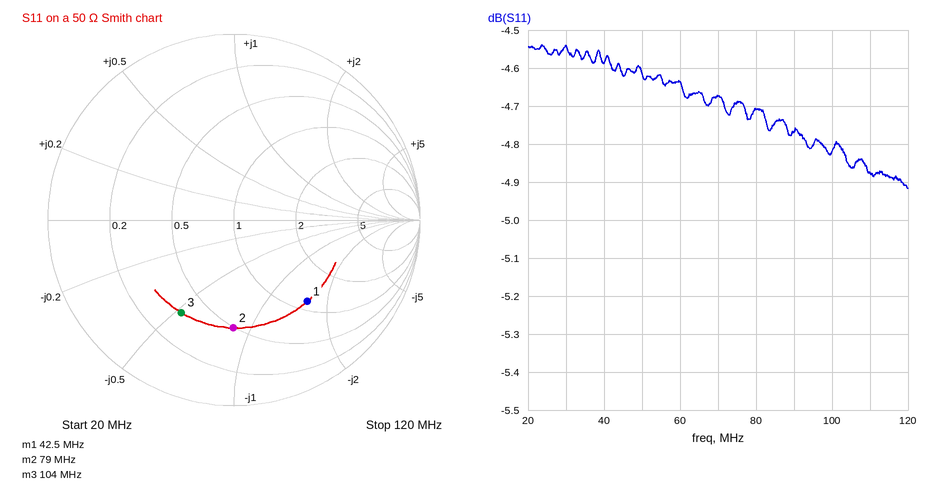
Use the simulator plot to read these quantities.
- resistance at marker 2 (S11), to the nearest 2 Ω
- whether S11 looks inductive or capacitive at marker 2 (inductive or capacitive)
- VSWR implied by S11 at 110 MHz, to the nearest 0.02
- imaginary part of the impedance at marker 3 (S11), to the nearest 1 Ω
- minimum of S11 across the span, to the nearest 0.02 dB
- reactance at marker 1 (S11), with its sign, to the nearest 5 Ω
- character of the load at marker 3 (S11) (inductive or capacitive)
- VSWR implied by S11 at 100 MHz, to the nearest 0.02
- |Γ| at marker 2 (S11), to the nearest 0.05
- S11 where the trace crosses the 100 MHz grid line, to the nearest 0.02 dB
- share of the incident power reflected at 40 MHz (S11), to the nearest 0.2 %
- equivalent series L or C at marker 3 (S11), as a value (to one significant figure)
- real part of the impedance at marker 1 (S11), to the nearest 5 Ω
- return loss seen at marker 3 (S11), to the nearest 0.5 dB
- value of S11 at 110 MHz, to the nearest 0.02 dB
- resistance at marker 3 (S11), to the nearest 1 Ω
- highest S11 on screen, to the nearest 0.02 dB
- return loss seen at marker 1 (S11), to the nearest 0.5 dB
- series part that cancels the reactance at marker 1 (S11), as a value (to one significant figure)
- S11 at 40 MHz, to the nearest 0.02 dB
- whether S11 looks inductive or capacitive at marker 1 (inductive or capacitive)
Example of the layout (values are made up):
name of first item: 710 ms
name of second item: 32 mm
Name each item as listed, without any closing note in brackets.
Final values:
resistance at marker 2 (S11), to the nearest 2 Ω: 24 Ω
whether S11 looks inductive or capacitive at marker 2: capacitive
VSWR implied by S11 at 110 MHz, to the nearest 0.02: 3.66
imaginary part of the impedance at marker 3 (S11), to the nearest 1 Ω: -26 Ω
minimum of S11 across the span, to the nearest 0.02 dB: -4.92 dB
reactance at marker 1 (S11), with its sign, to the nearest 5 Ω: -80 Ω
character of the load at marker 3 (S11): capacitive
VSWR implied by S11 at 100 MHz, to the nearest 0.02: 3.70
|Γ| at marker 2 (S11), to the nearest 0.05: 0.60
S11 where the trace crosses the 100 MHz grid line, to the nearest 0.02 dB: -4.82 dB
share of the incident power reflected at 40 MHz (S11), to the nearest 0.2 %: 34.8 %
equivalent series L or C at marker 3 (S11), as a value: 60 pF
real part of the impedance at marker 1 (S11), to the nearest 5 Ω: 60 Ω
return loss seen at marker 3 (S11), to the nearest 0.5 dB: 5.0 dB
value of S11 at 110 MHz, to the nearest 0.02 dB: -4.88 dB
resistance at marker 3 (S11), to the nearest 1 Ω: 18 Ω
highest S11 on screen, to the nearest 0.02 dB: -4.54 dB
return loss seen at marker 1 (S11), to the nearest 0.5 dB: 4.5 dB
series part that cancels the reactance at marker 1 (S11), as a value: 300 nH
S11 at 40 MHz, to the nearest 0.02 dB: -4.58 dB
whether S11 looks inductive or capacitive at marker 1: capacitive
